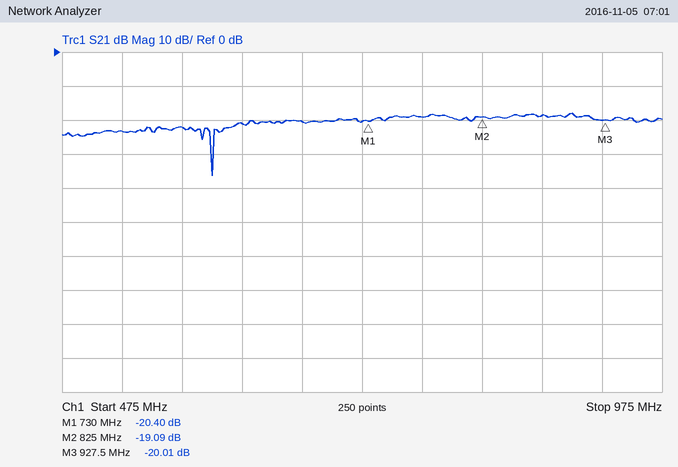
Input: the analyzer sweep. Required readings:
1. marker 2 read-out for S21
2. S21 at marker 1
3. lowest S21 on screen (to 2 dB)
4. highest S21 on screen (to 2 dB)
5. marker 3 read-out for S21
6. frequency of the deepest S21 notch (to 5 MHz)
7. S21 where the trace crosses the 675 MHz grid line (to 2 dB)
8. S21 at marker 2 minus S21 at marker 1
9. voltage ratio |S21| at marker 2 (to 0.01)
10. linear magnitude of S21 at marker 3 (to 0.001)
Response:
-19.09 dB
-20.40 dB
-36 dB
-18 dB
-20.01 dB
600 MHz
-20 dB
1.31 dB
0.11
0.100
